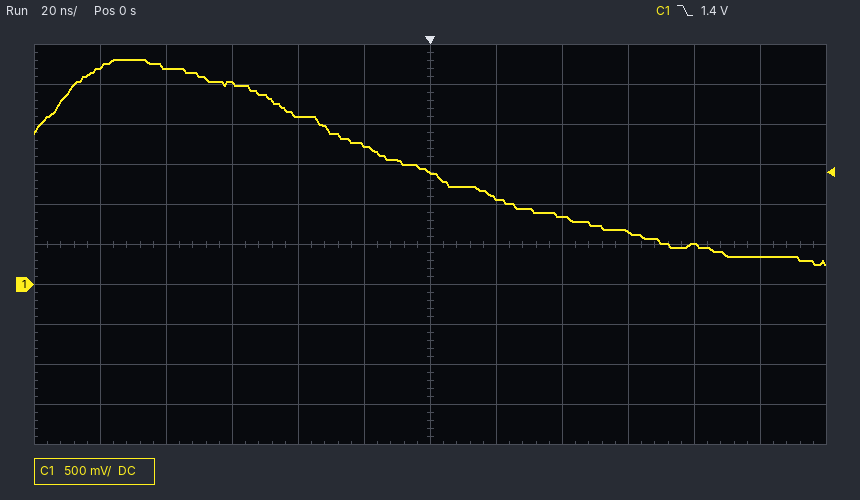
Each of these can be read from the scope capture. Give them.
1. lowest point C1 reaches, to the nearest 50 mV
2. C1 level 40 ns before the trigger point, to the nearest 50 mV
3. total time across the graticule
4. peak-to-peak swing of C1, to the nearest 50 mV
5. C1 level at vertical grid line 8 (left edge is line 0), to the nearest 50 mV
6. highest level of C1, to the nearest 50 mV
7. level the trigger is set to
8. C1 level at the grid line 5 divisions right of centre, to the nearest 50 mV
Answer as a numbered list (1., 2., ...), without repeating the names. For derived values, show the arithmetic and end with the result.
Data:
1. 250 mV
2. 2.10 V
3. 240 ns
4. 2.80 V − (250 mV) = 2.55 V
5. 850 mV
6. 2.80 V
7. 1.4 V
8. 350 mV
